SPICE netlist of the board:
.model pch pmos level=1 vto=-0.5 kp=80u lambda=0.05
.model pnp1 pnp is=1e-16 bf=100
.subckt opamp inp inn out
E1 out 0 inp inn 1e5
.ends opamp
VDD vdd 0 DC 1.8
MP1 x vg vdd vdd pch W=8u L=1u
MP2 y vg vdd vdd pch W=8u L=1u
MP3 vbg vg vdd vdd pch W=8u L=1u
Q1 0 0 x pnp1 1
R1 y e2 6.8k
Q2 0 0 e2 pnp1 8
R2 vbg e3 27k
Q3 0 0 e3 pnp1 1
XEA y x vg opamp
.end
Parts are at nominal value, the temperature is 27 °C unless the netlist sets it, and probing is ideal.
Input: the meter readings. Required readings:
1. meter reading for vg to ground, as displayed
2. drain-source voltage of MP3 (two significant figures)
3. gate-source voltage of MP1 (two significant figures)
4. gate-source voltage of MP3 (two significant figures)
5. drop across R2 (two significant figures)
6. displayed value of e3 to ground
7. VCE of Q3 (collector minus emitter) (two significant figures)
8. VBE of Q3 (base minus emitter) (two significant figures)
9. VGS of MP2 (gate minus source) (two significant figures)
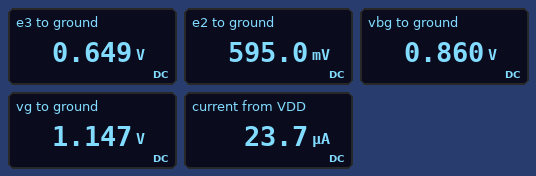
1.147 V
-940 mV
-650 mV
-650 mV
210 mV
0.649 V
-650 mV
-650 mV
-650 mV
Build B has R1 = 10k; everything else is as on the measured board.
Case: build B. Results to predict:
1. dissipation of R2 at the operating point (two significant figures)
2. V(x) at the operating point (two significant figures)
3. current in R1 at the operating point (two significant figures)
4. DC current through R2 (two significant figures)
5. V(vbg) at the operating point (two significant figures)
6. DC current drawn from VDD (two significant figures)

770 nW
640 mV
5.4 µA
5.3 µA
780 mV
16 µA
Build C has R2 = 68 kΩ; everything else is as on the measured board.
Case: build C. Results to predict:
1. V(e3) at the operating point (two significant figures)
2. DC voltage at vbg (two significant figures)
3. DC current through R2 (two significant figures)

650 mV
1.2 V
7.7 µA
